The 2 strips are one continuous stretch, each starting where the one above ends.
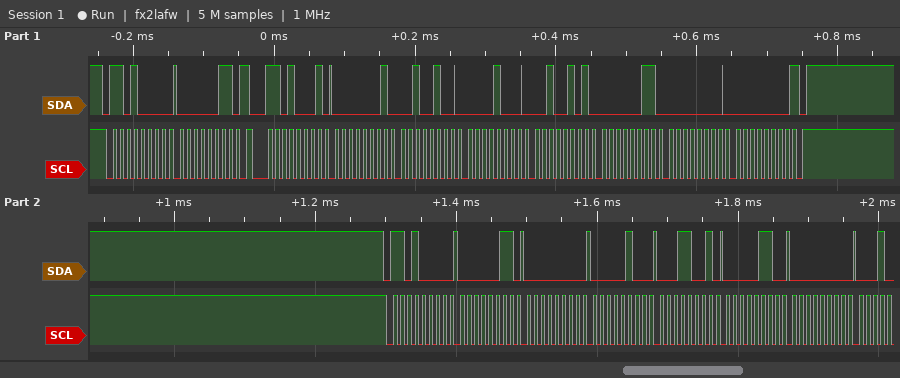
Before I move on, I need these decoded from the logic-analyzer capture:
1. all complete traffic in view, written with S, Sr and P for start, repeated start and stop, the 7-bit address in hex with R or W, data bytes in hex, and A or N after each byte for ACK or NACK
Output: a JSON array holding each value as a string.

["S 68W A 03 A Sr 68R A 01 A 24 A 08 A 25 A 03 A 00 A 00 N P S 68W A 03 A 00 A 04 A 19 A 06 A 00 A"]
